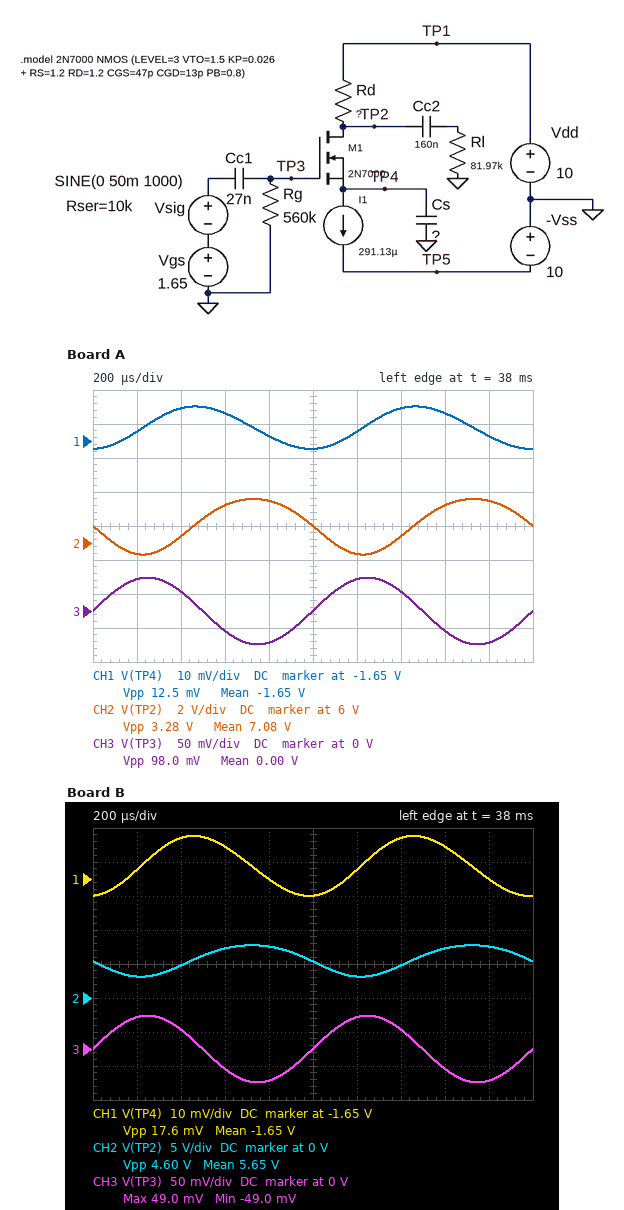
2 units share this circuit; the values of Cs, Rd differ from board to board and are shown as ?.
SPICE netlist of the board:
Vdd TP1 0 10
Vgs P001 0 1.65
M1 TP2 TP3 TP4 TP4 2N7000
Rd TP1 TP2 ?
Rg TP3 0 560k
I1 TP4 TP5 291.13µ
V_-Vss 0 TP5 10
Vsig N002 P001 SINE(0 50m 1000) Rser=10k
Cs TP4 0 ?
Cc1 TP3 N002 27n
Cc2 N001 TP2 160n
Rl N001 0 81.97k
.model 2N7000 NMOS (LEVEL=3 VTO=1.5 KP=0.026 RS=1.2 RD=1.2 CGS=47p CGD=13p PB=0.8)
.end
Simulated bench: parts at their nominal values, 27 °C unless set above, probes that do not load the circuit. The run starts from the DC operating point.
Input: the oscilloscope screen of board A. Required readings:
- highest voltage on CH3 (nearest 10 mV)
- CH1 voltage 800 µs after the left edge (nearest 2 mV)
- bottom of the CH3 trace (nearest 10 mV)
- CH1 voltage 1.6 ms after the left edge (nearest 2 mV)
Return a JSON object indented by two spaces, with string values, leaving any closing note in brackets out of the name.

{
  "highest voltage on CH3": "50 mV",
  "CH1 voltage 800 µs after the left edge": "-1.648 V",
  "bottom of the CH3 trace": "-50 mV",
  "CH1 voltage 1.6 ms after the left edge": "-1.642 V"
}
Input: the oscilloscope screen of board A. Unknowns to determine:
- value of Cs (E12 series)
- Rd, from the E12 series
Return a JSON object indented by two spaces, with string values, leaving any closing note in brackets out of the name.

{
  "value of Cs": "4.7 µF",
  "Rd, from the E12 series": "10 kΩ"
}
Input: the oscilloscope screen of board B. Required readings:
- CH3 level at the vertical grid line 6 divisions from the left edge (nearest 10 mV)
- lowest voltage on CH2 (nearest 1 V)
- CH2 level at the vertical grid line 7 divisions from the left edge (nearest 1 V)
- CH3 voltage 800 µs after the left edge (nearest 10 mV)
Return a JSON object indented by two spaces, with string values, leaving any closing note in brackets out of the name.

{
  "CH3 level at the vertical grid line 6 divisions from the left edge": "50 mV",
  "lowest voltage on CH2": "3 V",
  "CH2 level at the vertical grid line 7 divisions from the left edge": "5 V",
  "CH3 voltage 800 µs after the left edge": "-50 mV"
}
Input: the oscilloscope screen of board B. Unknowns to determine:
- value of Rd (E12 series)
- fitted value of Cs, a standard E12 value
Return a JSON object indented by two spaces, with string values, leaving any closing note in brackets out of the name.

{
  "value of Rd": "15 kΩ",
  "fitted value of Cs, a standard E12 value": "3.3 µF"
}
